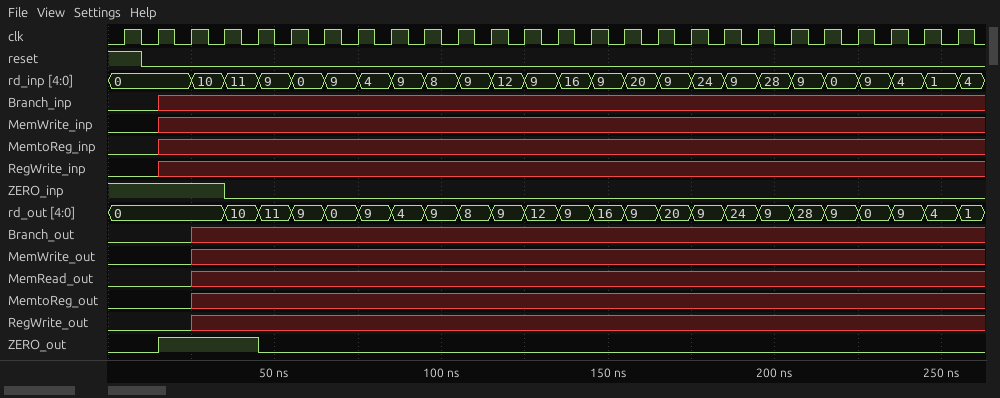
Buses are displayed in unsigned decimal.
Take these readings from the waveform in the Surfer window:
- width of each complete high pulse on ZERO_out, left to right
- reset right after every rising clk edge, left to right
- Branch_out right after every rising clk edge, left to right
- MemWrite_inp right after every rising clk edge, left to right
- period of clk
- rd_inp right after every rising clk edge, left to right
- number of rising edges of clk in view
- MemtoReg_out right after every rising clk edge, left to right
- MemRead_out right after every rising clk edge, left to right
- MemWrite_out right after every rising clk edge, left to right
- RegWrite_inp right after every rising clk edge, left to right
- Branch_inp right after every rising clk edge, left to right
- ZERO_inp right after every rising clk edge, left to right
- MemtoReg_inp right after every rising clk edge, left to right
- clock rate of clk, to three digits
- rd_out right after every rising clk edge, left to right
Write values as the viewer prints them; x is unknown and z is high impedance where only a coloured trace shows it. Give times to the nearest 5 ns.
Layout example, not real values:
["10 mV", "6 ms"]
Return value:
["30 ns", "1 0 0 0 0 0 0 0 0 0 0 0 0 0 0 0 0 0 0 0 0 0 0 0 0 0", "0 0 x x x x x x x x x x x x x x x x x x x x x x x x", "0 x x x x x x x x x x x x x x x x x x x x x x x x x", "10 ns", "0, 0, 10, 11, 9, 0, 9, 4, 9, 8, 9, 12, 9, 16, 9, 20, 9, 24, 9, 28, 9, 0, 9, 4, 1, 4", "26", "0 0 x x x x x x x x x x x x x x x x x x x x x x x x", "0 0 x x x x x x x x x x x x x x x x x x x x x x x x", "0 0 x x x x x x x x x x x x x x x x x x x x x x x x", "0 x x x x x x x x x x x x x x x x x x x x x x x x x", "0 x x x x x x x x x x x x x x x x x x x x x x x x x", "1 1 1 0 0 0 0 0 0 0 0 0 0 0 0 0 0 0 0 0 0 0 0 0 0 0", "0 x x x x x x x x x x x x x x x x x x x x x x x x x", "100 MHz", "0, 0, 0, 10, 11, 9, 0, 9, 4, 9, 8, 9, 12, 9, 16, 9, 20, 9, 24, 9, 28, 9, 0, 9, 4, 1"]
